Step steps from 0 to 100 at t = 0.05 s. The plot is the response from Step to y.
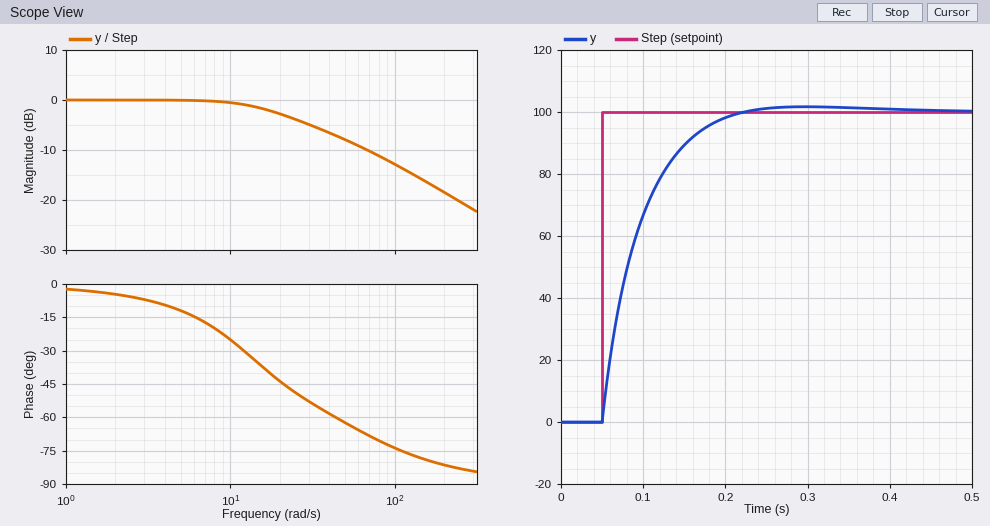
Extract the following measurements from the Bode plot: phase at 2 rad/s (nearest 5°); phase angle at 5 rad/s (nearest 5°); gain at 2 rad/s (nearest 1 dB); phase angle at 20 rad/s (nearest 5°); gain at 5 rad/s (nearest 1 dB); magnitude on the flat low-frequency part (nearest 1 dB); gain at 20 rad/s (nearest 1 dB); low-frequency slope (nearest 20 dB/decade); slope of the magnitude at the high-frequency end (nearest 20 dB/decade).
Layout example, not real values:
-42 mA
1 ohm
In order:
-5°
-10°
0 dB
-45°
0 dB
0 dB
-3 dB
0 dB/decade
-20 dB/decade
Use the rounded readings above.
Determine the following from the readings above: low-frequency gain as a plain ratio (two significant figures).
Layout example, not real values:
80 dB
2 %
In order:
1.0
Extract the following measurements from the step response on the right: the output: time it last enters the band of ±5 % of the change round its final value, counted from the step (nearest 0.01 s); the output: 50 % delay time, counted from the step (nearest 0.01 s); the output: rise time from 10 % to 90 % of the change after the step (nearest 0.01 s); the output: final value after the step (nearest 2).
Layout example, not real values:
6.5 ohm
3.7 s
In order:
0.13 s
0.03 s
0.10 s
100
